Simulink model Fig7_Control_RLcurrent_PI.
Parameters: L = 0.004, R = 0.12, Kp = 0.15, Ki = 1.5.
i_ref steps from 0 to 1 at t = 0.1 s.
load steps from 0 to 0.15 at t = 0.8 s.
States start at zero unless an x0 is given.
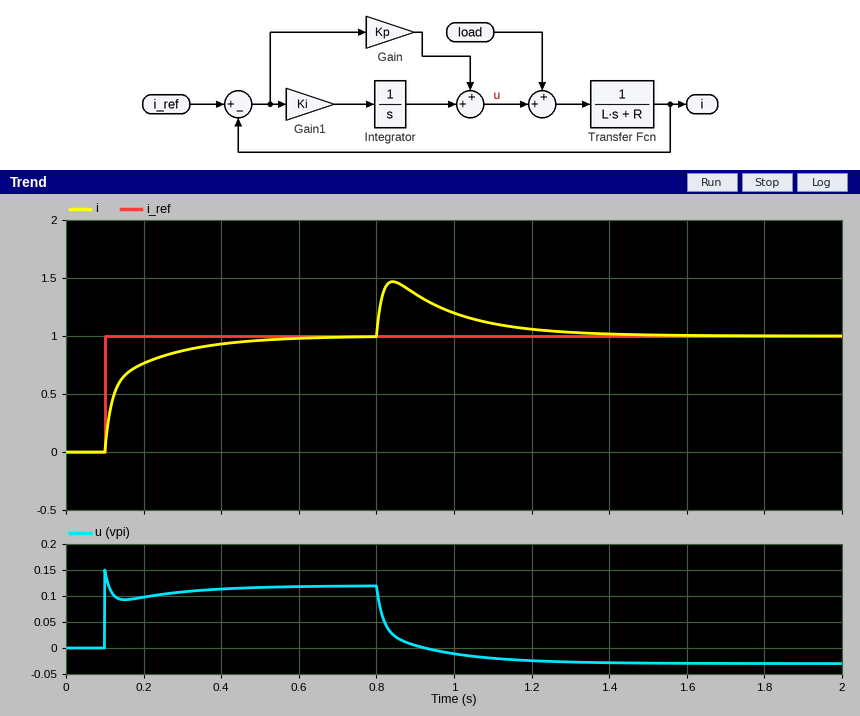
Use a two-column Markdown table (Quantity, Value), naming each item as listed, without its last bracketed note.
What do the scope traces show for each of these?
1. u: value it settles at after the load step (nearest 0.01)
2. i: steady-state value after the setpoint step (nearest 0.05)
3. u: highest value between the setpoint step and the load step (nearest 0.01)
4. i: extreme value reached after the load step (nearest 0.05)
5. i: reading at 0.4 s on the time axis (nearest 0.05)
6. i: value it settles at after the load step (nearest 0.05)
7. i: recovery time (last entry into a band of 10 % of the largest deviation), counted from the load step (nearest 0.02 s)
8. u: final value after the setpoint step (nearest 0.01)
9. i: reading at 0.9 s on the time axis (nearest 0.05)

| Quantity | Value |
|---|---|
| u: value it settles at after the load step | -0.03 |
| i: steady-state value after the setpoint step | 1.00 |
| u: highest value between the setpoint step and the load step | 0.15 |
| i: extreme value reached after the load step | 1.45 |
| i: reading at 0.4 s on the time axis | 0.95 |
| i: value it settles at after the load step | 1.00 |
| i: recovery time (last entry into a band of 10 % of the largest deviation), counted from the load step | 0.44 s |
| u: final value after the setpoint step | 0.12 |
| i: reading at 0.9 s on the time axis | 1.35 |
